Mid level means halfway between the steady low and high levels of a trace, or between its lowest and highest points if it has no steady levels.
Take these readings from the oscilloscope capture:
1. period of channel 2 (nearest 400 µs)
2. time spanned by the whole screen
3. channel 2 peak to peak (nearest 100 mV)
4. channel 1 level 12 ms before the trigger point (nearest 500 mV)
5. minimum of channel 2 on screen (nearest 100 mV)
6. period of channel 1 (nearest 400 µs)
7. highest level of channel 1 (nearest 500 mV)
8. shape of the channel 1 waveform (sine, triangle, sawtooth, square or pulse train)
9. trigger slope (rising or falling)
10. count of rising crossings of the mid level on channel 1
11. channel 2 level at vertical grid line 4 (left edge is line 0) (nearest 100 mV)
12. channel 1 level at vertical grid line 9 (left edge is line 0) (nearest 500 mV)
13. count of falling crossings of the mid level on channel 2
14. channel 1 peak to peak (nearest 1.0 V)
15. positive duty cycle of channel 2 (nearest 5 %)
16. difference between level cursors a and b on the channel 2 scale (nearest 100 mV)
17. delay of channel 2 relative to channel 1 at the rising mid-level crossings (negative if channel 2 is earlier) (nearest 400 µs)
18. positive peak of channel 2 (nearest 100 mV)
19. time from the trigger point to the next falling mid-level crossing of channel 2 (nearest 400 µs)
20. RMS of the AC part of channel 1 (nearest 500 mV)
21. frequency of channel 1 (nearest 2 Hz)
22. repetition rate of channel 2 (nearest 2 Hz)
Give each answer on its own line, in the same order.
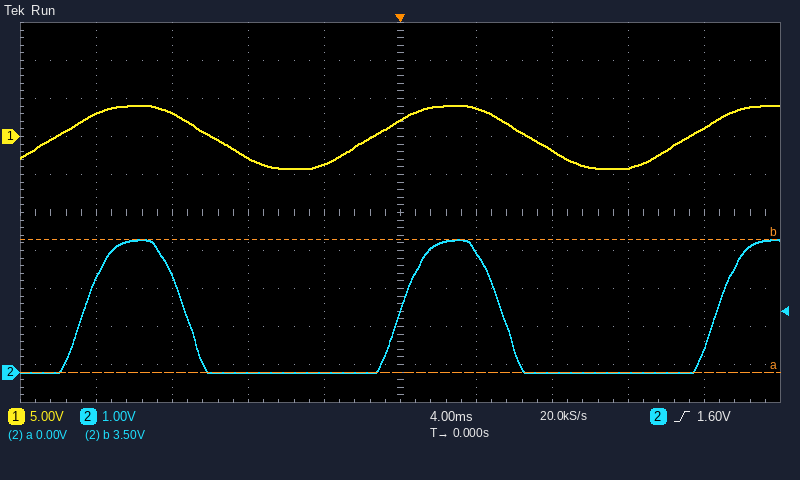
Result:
16.8 ms
40 ms
3.5 V
3.0 V
0.0 V
16.8 ms
4.0 V
sine
rising
3
0.0 V
1.0 V
2
8.0 V
30 %
3.5 V
+1.6 ms
3.5 V
5.2 ms
3.0 V
60 Hz
60 Hz
